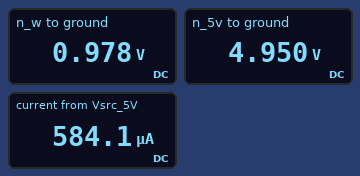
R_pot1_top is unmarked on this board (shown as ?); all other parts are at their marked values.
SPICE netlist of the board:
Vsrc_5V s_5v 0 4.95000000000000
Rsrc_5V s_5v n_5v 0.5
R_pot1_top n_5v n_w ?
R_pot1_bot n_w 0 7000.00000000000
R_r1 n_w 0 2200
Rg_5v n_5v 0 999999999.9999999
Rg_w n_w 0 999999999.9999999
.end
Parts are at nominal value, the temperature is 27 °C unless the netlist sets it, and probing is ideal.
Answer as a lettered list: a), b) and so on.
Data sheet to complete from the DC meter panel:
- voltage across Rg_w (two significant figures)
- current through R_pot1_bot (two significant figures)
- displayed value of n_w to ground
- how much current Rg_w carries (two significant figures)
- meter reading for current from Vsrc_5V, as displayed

a) 980 mV
b) 140 µA
c) 0.978 V
d) 980 pA
e) 584.1 µA
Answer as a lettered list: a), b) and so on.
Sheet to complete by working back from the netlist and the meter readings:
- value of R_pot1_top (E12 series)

a) 6.8 kΩ
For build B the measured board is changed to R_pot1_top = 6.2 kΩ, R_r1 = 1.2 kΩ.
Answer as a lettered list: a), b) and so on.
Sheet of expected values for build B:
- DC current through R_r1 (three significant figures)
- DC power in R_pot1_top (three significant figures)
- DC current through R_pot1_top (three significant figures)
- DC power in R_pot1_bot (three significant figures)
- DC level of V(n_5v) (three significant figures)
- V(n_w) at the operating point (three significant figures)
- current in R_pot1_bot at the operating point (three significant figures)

a) 585 µA
b) 2.91 mW
c) 685 µA
d) 70.4 µW
e) 4.95 V
f) 702 mV
g) 100 µA
